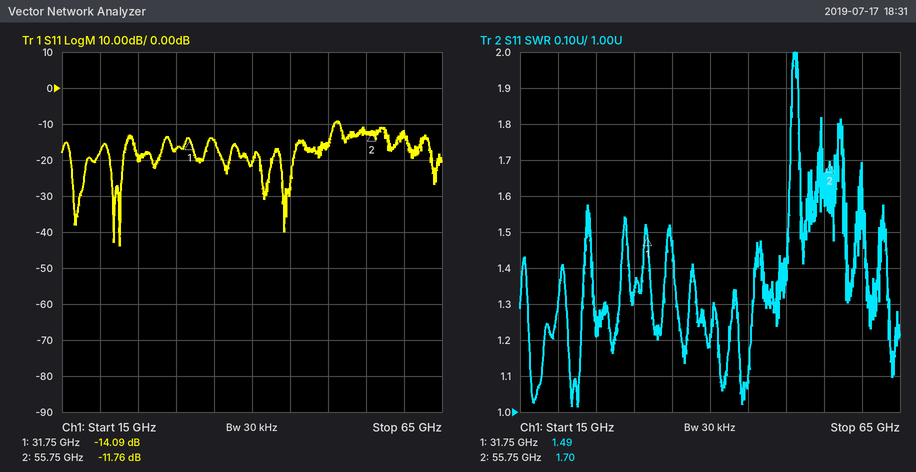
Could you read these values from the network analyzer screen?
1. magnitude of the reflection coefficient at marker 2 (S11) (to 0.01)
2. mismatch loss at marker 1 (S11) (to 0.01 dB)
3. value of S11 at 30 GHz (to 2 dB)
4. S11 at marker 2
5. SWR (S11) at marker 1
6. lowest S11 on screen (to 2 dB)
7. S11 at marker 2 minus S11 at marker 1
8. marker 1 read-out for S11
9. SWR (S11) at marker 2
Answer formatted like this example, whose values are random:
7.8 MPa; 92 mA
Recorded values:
0.26; 0.17 dB; -16 dB; -11.76 dB; 1.49; -44 dB; 2.33 dB; -14.09 dB; 1.70
